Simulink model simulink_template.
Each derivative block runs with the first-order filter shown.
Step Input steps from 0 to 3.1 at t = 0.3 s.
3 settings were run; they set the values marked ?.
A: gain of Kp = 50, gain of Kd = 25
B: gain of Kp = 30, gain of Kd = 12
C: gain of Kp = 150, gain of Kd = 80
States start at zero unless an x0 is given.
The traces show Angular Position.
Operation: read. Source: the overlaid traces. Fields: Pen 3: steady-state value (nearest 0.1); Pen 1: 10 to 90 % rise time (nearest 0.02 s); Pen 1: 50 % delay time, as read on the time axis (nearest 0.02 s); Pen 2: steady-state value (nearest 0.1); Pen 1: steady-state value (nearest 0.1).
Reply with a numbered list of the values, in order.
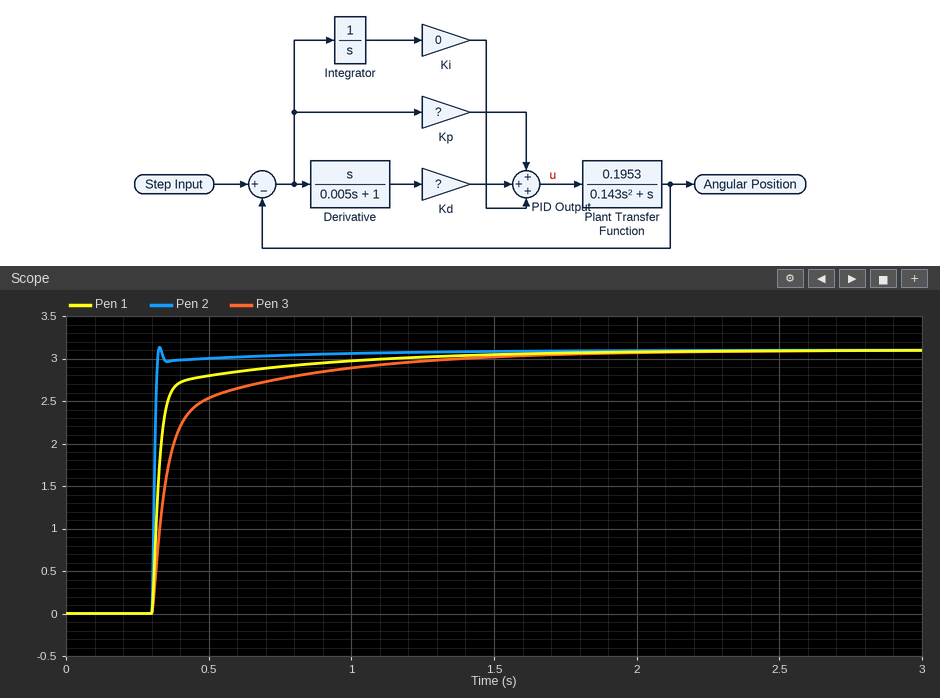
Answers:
1. 3.1
2. 0.18 s
3. 0.32 s
4. 3.1
5. 3.1
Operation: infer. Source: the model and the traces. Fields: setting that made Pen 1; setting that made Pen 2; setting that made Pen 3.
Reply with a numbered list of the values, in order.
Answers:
1. A
2. C
3. B
